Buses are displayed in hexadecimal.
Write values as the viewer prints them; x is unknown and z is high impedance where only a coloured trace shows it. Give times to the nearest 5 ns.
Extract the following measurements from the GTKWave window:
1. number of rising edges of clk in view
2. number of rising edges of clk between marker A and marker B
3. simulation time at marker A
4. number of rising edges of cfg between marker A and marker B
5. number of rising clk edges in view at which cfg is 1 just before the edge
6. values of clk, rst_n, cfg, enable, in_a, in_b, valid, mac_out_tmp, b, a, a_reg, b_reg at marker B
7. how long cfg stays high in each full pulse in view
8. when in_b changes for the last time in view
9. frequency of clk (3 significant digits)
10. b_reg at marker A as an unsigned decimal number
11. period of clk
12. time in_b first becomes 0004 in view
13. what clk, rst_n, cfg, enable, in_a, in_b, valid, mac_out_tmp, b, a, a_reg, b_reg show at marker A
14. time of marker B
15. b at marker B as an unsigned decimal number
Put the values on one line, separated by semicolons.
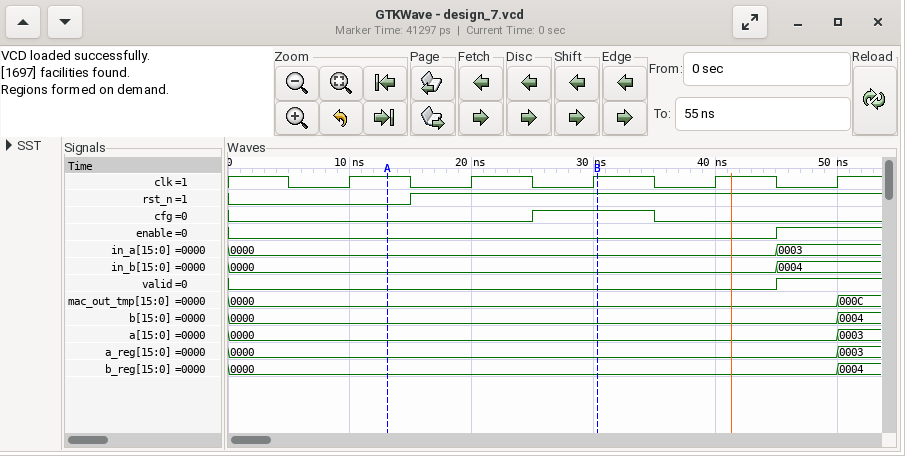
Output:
5; 2; 15 ns; 1; 1; clk=1, rst_n=1, cfg=1, enable=0, in_a=0000, in_b=0000, valid=0, mac_out_tmp=0000, b=0000, a=0000, a_reg=0000, b_reg=0000; 10 ns; 45 ns; 100 MHz; 0; 10 ns; 45 ns; clk=1, rst_n=0, cfg=0, enable=0, in_a=0000, in_b=0000, valid=0, mac_out_tmp=0000, b=0000, a=0000, a_reg=0000, b_reg=0000; 30 ns; 0
